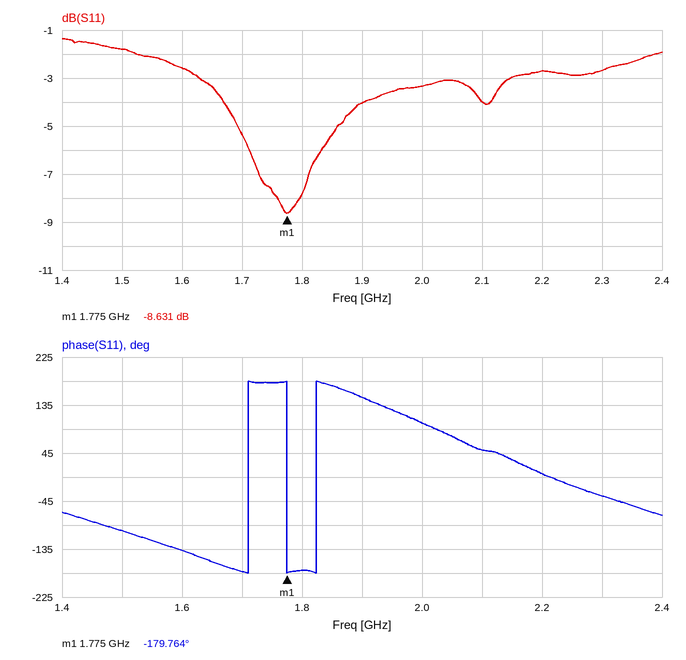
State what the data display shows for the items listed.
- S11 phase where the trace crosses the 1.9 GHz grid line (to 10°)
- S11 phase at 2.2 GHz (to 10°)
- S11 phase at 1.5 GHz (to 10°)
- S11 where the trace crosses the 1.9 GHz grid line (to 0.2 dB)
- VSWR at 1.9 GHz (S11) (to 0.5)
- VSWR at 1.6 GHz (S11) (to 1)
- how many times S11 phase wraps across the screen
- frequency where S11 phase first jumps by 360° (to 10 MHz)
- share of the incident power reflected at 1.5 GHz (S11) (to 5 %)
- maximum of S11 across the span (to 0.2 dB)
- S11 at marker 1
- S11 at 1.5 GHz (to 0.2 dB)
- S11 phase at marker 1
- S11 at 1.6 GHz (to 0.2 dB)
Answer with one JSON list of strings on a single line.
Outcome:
["150°", "10°", "-100°", "-4.0 dB", "4.5", "7", "3", "1.71 GHz", "65 %", "-1.4 dB", "-8.631 dB", "-1.8 dB", "-179.764°", "-2.6 dB"]
